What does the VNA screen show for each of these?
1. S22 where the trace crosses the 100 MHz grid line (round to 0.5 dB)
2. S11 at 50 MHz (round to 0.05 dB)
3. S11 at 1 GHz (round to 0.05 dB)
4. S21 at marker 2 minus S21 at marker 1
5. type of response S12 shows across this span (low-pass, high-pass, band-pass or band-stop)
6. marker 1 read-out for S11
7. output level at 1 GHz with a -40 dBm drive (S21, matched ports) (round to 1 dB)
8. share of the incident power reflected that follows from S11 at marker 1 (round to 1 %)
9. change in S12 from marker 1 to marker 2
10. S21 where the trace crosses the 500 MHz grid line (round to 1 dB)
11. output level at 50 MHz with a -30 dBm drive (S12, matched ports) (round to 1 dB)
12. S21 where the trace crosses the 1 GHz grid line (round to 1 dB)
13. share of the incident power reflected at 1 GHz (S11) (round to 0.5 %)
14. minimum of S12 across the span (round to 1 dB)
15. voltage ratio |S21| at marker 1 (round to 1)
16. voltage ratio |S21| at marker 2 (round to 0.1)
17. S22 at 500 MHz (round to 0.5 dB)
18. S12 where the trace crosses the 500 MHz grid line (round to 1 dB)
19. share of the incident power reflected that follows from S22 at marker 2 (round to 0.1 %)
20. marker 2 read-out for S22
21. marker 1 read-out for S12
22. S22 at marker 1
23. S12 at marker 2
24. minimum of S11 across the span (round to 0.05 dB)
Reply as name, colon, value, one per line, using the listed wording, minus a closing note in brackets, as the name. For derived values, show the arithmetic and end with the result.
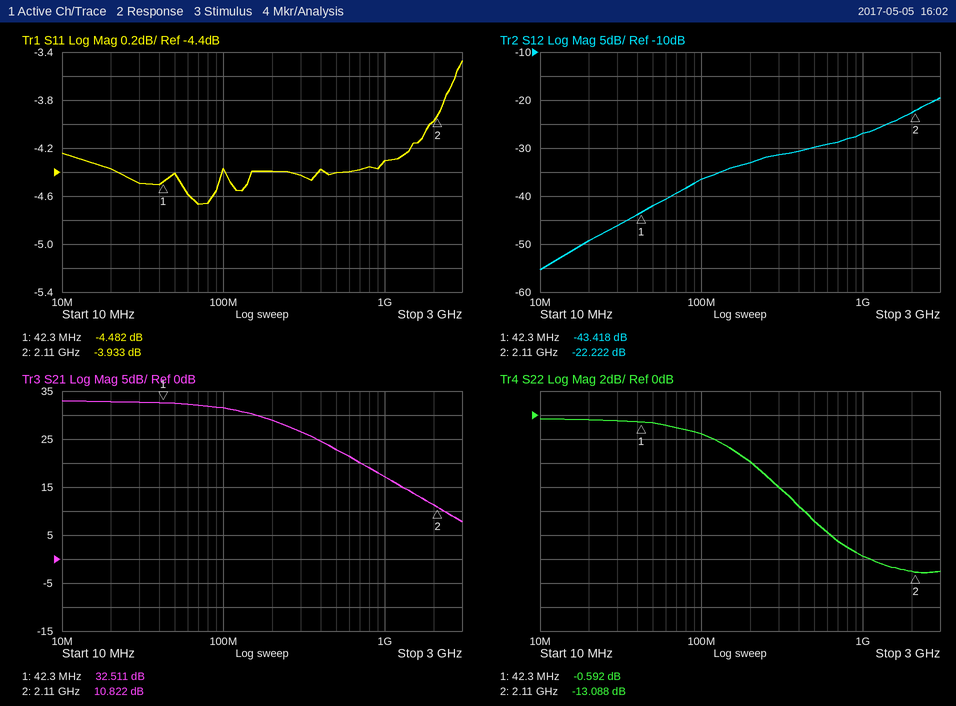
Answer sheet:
S22 where the trace crosses the 100 MHz grid line: -1.5 dB
S11 at 50 MHz: -4.40 dB
S11 at 1 GHz: -4.30 dB
S21 at marker 2 minus S21 at marker 1: 10.822 − (32.511) = -21.689 dB
type of response S12 shows across this span: high-pass
marker 1 read-out for S11: -4.482 dB
output level at 1 GHz with a -40 dBm drive (S21, matched ports): -40 dBm + (17 dB) = -23 dBm
share of the incident power reflected that follows from S11 at marker 1: 10^(-4.482/10) ≈ 36 %
change in S12 from marker 1 to marker 2: -22.222 − (-43.418) = 21.196 dB
S21 where the trace crosses the 500 MHz grid line: 23 dB
output level at 50 MHz with a -30 dBm drive (S12, matched ports): -30 dBm + (-42 dB) = -72 dBm
S21 where the trace crosses the 1 GHz grid line: 17 dB
share of the incident power reflected at 1 GHz (S11): 10^(-4.3/10) ≈ 37.2 %, so 37.0 % to the nearest 0.5 %
minimum of S12 across the span: -55 dB
voltage ratio |S21| at marker 1: 10^(32.511/20) ≈ 42
voltage ratio |S21| at marker 2: 10^(10.822/20) ≈ 3.5
S22 at 500 MHz: -9.0 dB
S12 where the trace crosses the 500 MHz grid line: -30 dB
share of the incident power reflected that follows from S22 at marker 2: 10^(-13.088/10) ≈ 4.9 %
marker 2 read-out for S22: -13.088 dB
marker 1 read-out for S12: -43.418 dB
S22 at marker 1: -0.592 dB
S12 at marker 2: -22.222 dB
minimum of S11 across the span: -4.65 dB
